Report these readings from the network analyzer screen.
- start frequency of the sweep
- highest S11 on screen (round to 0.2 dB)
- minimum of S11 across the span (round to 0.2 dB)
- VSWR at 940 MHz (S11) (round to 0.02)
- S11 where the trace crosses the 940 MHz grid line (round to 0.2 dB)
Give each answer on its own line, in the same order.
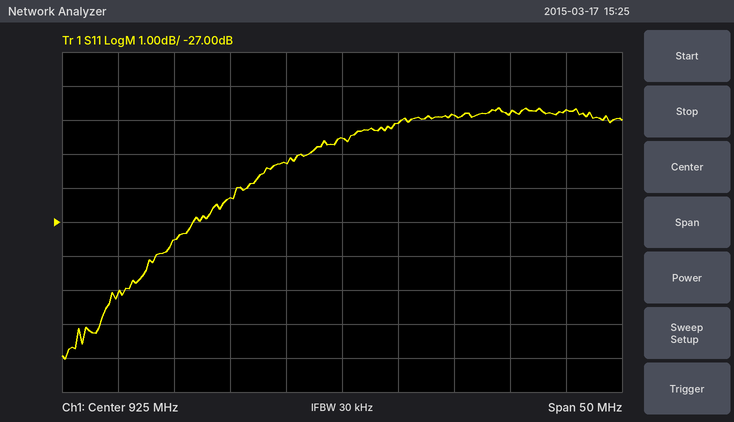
900 MHz
-23.6 dB
-31.0 dB
1.14
-23.8 dB
